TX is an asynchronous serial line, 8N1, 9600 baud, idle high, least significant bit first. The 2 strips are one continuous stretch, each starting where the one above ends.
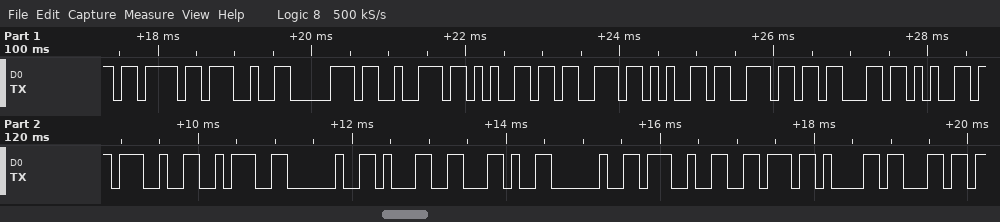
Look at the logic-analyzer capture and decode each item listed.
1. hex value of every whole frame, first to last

7B 27 70 72 65 73 65 6E 63 65 27 3A 20 31 2C 20 27 76 61 6C
